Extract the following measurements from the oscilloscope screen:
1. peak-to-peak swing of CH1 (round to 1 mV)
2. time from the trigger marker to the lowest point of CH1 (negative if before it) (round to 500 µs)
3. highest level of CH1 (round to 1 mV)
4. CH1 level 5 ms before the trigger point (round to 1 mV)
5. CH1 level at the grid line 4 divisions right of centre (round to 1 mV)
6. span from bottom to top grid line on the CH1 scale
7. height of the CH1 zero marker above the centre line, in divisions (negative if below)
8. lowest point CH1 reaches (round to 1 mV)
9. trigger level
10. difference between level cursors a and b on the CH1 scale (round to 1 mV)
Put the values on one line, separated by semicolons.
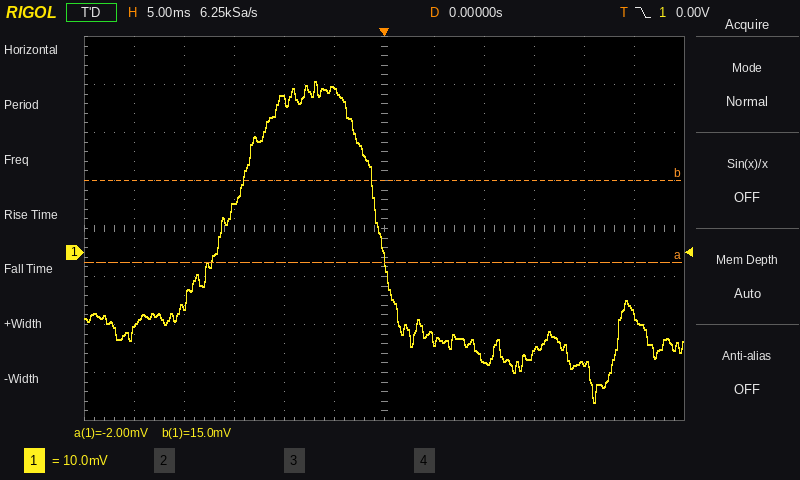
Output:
67 mV; +21.0 ms; 36 mV; 34 mV; -23 mV; 80 mV; -0.5 div; -31 mV; 0.00 V; 17 mV
